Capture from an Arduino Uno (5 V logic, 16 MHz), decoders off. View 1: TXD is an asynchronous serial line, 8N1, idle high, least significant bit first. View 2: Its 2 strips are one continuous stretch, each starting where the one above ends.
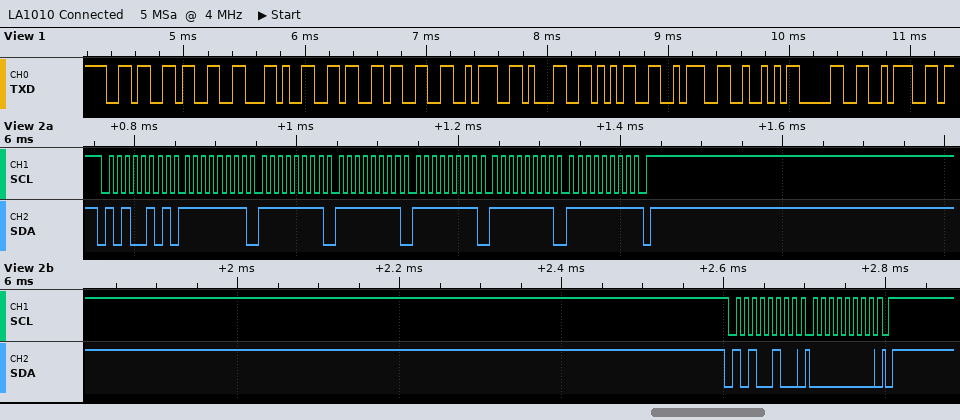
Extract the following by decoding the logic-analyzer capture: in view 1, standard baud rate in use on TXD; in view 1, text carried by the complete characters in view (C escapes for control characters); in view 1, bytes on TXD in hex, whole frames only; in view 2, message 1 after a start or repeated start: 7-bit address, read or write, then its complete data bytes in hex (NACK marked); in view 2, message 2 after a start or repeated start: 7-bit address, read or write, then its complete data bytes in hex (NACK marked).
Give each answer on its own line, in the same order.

19200 baud
"63,63:15:R0:"
36 33 2C 36 33 3A 31 35 3A 52 30 3A
0x52 read: FF FF FF FF FF FF NACK
0x52 write: 00
